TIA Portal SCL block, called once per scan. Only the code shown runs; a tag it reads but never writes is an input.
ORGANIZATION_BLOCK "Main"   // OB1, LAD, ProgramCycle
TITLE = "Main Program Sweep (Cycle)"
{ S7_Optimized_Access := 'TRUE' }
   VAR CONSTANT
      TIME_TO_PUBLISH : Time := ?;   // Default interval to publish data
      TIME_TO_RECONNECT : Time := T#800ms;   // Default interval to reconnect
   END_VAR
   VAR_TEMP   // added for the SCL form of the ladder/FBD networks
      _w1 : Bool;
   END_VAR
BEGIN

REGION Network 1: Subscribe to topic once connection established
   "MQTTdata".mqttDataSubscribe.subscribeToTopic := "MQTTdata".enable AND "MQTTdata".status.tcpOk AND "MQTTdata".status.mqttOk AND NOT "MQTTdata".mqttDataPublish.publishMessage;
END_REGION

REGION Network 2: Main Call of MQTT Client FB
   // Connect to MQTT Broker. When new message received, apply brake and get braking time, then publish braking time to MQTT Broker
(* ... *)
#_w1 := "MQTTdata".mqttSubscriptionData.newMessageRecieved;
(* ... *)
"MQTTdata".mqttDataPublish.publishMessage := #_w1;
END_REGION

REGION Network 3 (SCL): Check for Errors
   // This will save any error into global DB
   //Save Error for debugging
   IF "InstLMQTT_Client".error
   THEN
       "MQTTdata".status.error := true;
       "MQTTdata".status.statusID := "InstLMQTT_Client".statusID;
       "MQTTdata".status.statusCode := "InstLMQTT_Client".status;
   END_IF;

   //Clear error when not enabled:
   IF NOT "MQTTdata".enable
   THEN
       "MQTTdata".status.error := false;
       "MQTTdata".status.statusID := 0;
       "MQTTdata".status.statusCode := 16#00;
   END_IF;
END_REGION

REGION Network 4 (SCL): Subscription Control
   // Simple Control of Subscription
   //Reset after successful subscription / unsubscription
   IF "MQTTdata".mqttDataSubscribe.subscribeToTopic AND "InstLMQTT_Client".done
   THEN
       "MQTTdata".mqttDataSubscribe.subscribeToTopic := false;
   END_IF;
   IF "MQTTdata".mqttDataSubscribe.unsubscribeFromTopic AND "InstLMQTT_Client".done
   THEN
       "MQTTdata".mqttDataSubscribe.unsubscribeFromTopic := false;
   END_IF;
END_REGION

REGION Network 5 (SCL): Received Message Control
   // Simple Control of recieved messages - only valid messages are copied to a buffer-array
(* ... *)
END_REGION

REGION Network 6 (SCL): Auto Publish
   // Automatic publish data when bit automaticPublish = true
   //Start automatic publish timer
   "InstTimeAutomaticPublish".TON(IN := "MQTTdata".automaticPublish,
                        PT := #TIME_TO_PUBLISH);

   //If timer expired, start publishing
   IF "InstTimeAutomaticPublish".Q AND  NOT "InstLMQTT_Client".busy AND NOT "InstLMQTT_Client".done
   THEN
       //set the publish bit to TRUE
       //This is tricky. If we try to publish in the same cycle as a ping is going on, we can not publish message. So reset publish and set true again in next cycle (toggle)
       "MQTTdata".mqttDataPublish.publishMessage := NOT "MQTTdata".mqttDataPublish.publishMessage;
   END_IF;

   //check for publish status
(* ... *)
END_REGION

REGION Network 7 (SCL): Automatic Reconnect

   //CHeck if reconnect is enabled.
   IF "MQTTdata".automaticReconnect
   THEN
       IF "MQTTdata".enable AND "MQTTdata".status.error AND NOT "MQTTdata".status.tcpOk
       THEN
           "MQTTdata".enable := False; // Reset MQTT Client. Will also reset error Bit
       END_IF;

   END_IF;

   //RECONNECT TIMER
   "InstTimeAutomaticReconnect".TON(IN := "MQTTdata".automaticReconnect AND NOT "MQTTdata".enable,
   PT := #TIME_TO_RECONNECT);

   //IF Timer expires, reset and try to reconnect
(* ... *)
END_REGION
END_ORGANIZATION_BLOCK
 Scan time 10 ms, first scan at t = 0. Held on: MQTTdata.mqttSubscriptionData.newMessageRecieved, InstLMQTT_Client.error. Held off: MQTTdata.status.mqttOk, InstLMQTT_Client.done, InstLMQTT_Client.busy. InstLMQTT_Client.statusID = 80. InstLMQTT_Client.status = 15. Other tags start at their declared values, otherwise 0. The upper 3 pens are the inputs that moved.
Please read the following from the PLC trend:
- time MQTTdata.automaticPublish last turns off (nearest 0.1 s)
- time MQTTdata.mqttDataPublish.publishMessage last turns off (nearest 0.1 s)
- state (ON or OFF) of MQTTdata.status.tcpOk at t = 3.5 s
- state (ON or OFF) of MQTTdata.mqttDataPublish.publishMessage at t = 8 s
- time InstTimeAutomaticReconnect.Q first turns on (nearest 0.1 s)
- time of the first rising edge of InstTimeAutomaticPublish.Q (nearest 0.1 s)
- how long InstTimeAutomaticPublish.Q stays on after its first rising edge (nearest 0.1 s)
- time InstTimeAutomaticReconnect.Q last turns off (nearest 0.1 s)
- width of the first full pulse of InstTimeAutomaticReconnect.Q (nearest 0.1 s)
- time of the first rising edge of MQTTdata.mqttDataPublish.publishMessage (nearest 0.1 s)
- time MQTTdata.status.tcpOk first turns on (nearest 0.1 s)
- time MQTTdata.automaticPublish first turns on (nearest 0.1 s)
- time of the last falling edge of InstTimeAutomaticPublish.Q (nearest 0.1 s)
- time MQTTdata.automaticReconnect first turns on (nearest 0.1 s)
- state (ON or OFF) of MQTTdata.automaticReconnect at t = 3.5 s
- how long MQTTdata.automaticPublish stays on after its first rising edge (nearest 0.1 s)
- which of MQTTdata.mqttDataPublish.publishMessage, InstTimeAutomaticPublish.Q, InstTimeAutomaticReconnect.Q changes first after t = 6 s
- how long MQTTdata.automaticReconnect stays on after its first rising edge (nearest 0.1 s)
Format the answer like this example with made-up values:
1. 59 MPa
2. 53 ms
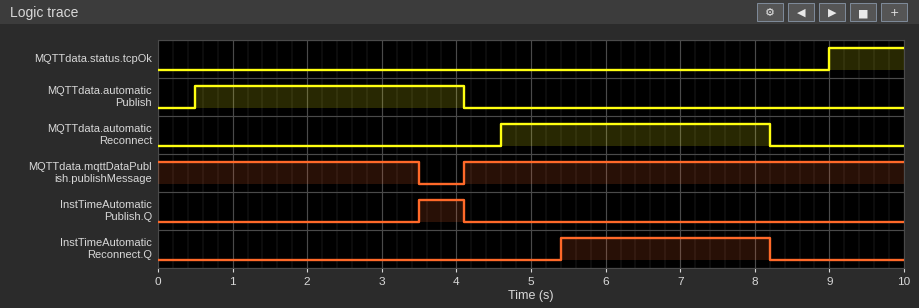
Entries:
1. 4.1 s
2. 3.5 s
3. OFF
4. ON
5. 5.4 s
6. 3.5 s
7. 0.6 s
8. 8.2 s
9. 2.8 s
10. 4.1 s
11. 9.0 s
12. 0.5 s
13. 4.1 s
14. 4.6 s
15. OFF
16. 3.6 s
17. InstTimeAutomaticReconnect.Q
18. 3.6 s
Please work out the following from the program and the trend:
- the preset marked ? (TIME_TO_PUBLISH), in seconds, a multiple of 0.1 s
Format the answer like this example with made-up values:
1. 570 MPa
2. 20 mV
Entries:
1. 3.0 s
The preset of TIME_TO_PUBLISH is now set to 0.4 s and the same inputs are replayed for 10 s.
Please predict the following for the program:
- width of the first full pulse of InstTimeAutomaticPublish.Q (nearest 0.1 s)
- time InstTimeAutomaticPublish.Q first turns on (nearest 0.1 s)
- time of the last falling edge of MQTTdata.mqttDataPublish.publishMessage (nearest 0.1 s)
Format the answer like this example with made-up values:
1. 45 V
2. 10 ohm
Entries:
1. 3.2 s
2. 0.9 s
3. 0.9 s
